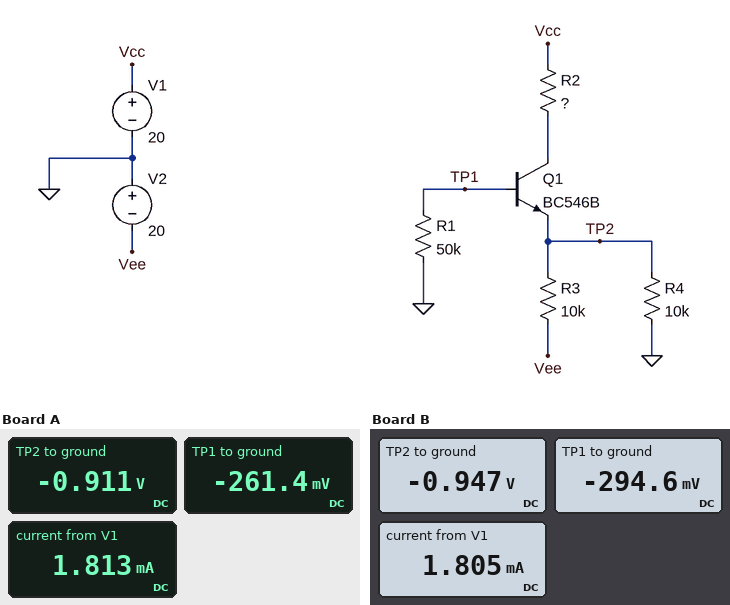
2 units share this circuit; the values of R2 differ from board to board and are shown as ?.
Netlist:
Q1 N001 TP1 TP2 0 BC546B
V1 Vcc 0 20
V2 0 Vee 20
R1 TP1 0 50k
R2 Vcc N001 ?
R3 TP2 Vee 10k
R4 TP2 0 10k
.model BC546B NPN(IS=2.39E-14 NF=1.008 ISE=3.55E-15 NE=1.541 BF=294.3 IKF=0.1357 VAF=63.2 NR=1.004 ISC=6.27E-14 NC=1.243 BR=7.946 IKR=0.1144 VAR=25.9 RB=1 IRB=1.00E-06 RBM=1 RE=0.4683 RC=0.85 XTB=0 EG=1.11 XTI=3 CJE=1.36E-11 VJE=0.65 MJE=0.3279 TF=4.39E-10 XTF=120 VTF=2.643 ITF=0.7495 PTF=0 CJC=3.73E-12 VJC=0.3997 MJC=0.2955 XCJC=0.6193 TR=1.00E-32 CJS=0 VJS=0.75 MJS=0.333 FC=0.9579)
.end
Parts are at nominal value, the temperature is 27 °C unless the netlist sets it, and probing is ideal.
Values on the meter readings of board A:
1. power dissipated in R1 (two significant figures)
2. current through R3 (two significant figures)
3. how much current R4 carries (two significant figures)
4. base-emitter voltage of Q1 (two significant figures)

1.4 µW
1.9 mA
91 µA
650 mV
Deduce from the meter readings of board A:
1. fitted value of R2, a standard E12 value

3.3 kΩ
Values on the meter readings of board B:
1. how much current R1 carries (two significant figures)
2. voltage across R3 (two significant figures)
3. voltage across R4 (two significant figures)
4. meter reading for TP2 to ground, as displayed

5.9 µA
19 V
950 mV
-0.947 V
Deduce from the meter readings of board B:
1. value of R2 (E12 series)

8.2 kΩ
